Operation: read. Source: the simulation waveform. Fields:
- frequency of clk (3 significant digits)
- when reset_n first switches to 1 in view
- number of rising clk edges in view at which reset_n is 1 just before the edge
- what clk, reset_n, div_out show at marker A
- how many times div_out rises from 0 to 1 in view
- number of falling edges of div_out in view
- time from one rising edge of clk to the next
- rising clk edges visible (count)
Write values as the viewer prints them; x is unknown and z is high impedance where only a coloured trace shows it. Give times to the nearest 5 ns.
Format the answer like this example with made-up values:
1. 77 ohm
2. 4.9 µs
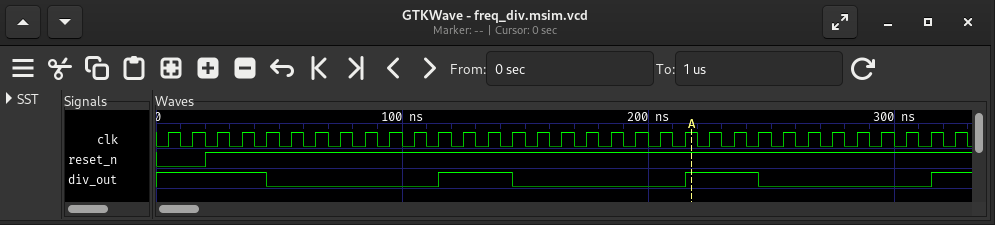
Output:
1. 100 MHz
2. 20 ns
3. 31
4. clk=1, reset_n=1, div_out=1
5. 3
6. 3
7. 10 ns
8. 33
